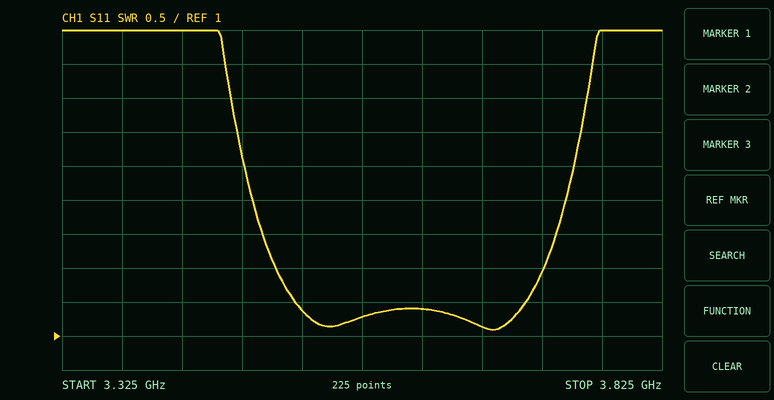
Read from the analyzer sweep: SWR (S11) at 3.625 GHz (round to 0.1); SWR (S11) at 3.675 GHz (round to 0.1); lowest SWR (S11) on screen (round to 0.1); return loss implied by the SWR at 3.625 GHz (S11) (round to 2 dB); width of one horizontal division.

1.4
1.1
1.1
16 dB
50 MHz
